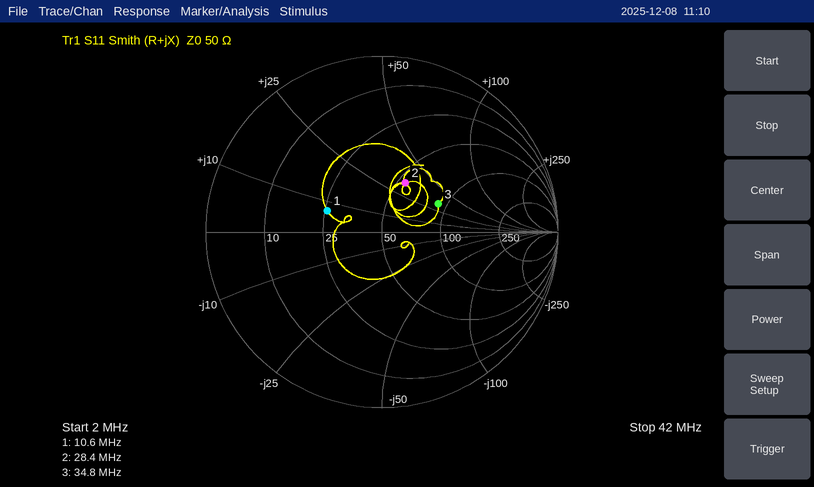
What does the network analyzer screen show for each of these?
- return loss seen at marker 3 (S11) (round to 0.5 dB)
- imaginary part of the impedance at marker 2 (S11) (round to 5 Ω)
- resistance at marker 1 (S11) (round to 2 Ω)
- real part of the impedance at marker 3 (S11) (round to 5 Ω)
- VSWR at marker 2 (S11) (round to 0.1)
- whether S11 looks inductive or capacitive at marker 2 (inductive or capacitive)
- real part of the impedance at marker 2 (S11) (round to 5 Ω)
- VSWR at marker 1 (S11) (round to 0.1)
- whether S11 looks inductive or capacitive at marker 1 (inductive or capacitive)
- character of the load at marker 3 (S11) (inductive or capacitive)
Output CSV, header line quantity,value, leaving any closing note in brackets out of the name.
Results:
quantity,value
return loss seen at marker 3 (S11),9.0 dB
imaginary part of the impedance at marker 2 (S11),+35 Ω
resistance at marker 1 (S11),26 Ω
real part of the impedance at marker 3 (S11),90 Ω
VSWR at marker 2 (S11),1.9
whether S11 looks inductive or capacitive at marker 2,inductive
real part of the impedance at marker 2 (S11),55 Ω
VSWR at marker 1 (S11),2.0
whether S11 looks inductive or capacitive at marker 1,inductive
character of the load at marker 3 (S11),inductive
